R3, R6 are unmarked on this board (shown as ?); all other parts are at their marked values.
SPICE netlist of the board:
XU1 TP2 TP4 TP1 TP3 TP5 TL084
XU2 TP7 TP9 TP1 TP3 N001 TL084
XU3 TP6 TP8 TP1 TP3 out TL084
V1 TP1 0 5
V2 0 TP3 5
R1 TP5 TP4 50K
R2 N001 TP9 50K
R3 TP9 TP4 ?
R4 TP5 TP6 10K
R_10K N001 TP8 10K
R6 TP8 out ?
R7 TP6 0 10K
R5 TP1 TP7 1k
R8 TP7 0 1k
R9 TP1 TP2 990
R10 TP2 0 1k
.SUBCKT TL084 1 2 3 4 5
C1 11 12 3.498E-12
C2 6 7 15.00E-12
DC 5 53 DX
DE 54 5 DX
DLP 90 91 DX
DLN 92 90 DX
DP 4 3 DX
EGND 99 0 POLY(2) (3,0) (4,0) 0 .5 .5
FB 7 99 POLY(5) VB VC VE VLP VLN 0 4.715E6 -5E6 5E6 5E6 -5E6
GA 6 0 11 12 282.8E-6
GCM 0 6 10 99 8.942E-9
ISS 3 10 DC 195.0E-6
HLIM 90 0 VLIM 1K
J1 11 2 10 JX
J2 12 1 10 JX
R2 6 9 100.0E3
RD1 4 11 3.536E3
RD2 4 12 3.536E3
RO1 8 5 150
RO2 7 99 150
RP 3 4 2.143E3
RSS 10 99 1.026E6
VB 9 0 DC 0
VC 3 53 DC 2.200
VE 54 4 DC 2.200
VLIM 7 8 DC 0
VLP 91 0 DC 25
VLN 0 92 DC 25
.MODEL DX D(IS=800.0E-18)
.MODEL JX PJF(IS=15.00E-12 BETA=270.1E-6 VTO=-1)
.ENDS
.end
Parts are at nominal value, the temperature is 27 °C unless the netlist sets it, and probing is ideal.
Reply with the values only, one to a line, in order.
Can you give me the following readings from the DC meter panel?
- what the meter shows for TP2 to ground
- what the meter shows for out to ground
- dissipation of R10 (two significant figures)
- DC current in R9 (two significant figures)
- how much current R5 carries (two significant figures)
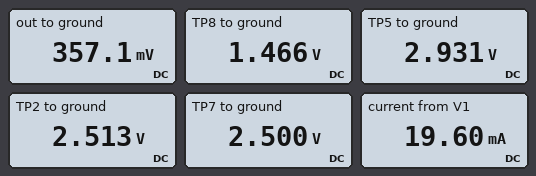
2.513 V
357.1 mV
6.3 mW
2.5 mA
2.5 mA
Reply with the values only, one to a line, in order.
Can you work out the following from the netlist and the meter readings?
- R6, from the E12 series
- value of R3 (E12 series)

18 kΩ
1.5 kΩ
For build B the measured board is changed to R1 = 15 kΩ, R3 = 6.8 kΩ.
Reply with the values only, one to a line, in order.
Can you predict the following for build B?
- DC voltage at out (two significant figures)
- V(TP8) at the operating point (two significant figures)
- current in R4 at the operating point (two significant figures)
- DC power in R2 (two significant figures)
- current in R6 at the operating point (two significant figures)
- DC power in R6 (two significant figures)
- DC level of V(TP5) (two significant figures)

-780 mV
1.3 V
130 µA
170 nW
110 µA
230 µW
2.5 V
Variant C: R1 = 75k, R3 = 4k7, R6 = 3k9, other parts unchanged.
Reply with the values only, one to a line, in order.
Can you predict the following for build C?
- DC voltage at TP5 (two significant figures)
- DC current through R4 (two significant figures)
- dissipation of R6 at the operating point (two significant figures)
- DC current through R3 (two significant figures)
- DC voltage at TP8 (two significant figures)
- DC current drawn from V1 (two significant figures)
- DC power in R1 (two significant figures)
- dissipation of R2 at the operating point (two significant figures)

2.7 V
140 µA
40 µW
2.7 µA
1.4 V
20 mA
540 nW
360 nW
